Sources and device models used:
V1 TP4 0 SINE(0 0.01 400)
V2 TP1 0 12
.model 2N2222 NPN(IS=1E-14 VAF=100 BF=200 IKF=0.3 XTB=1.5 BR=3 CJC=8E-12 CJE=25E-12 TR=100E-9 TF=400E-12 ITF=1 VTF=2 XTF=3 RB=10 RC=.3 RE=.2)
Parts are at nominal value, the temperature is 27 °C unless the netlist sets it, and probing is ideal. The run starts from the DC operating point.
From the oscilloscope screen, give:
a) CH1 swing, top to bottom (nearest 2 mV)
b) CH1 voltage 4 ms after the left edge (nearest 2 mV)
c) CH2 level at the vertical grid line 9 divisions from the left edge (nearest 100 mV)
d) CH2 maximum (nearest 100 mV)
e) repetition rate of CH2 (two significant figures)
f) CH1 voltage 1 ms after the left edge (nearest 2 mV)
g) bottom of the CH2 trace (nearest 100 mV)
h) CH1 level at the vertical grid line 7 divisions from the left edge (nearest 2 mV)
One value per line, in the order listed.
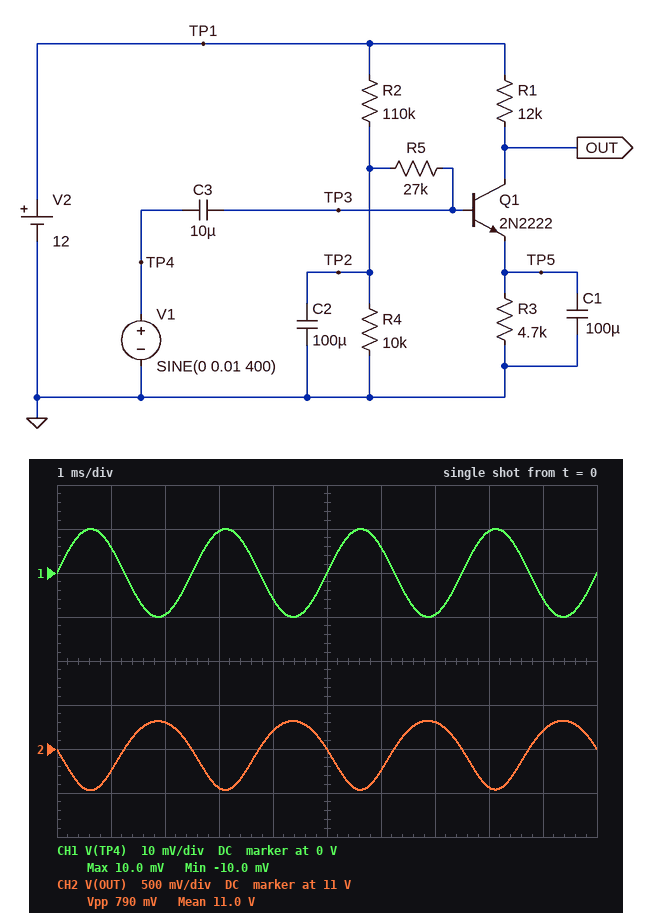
20 mV
-6 mV
11.2 V
11.3 V
400 Hz
6 mV
10.5 V
-10 mV
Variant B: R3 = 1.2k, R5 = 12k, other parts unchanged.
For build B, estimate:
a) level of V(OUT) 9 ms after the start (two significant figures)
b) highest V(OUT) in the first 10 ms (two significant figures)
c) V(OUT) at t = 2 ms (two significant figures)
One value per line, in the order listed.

9.3 V
9.7 V
9.6 V
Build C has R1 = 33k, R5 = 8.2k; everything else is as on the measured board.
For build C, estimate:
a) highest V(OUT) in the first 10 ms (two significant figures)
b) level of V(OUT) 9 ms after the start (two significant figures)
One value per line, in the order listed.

10 V
9.8 V
